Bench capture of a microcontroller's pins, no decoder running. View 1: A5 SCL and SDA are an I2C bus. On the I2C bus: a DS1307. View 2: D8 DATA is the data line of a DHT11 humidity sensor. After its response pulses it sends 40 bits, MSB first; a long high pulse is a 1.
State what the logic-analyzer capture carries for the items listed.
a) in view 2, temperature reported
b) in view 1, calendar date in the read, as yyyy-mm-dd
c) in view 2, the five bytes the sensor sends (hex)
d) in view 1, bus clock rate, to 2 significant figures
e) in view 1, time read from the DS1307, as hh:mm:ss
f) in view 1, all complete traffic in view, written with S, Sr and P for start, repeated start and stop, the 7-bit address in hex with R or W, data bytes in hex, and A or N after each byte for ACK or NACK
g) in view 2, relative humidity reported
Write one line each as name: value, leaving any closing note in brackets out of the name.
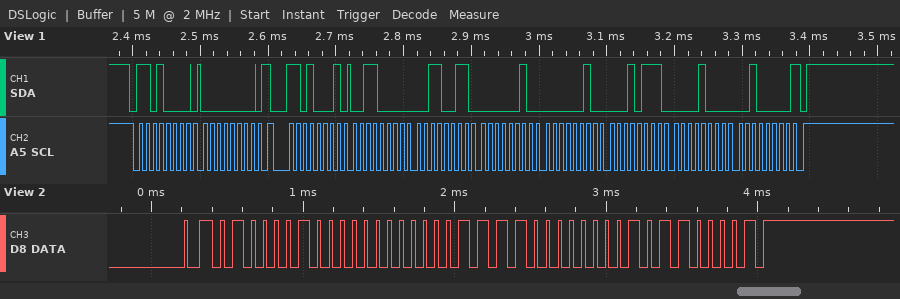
in view 2, temperature reported: 30.1 °C
in view 1, calendar date in the read, as yyyy-mm-dd: 2020-08-17
in view 2, the five bytes the sensor sends: 42 00 1E 01 61
in view 1, bus clock rate, to 2 significant figures: 100 kHz
in view 1, time read from the DS1307, as hh:mm:ss: 02:33:30
in view 1, all complete traffic in view, written with S, Sr and P for start, repeated start and stop, the 7-bit address in hex with R or W, data bytes in hex, and A or N after each byte for ACK or NACK: S 68W A 00 A Sr 68R A 30 A 33 A 02 A 02 A 17 A 08 A 20 N P
in view 2, relative humidity reported: 66 %
